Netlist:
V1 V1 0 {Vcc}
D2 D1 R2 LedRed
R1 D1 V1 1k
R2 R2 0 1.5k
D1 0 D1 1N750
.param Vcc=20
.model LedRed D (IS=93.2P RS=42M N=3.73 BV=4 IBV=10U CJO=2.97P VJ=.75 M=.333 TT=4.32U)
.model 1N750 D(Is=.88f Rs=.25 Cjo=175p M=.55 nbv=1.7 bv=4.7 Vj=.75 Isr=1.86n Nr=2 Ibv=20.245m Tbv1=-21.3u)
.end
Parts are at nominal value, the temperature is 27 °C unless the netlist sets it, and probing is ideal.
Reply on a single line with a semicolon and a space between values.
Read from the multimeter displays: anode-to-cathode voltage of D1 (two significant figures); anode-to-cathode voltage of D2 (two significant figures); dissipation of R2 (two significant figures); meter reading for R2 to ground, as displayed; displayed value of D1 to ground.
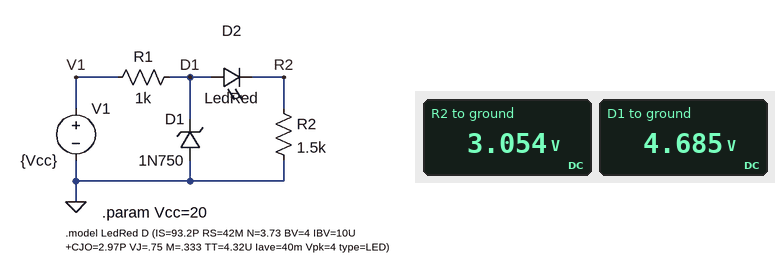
-4.7 V; 1.6 V; 6.2 mW; 3.054 V; 4.685 V
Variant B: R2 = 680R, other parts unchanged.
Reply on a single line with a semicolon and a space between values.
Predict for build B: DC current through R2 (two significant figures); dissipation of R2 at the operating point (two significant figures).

4.4 mA; 13 mW
